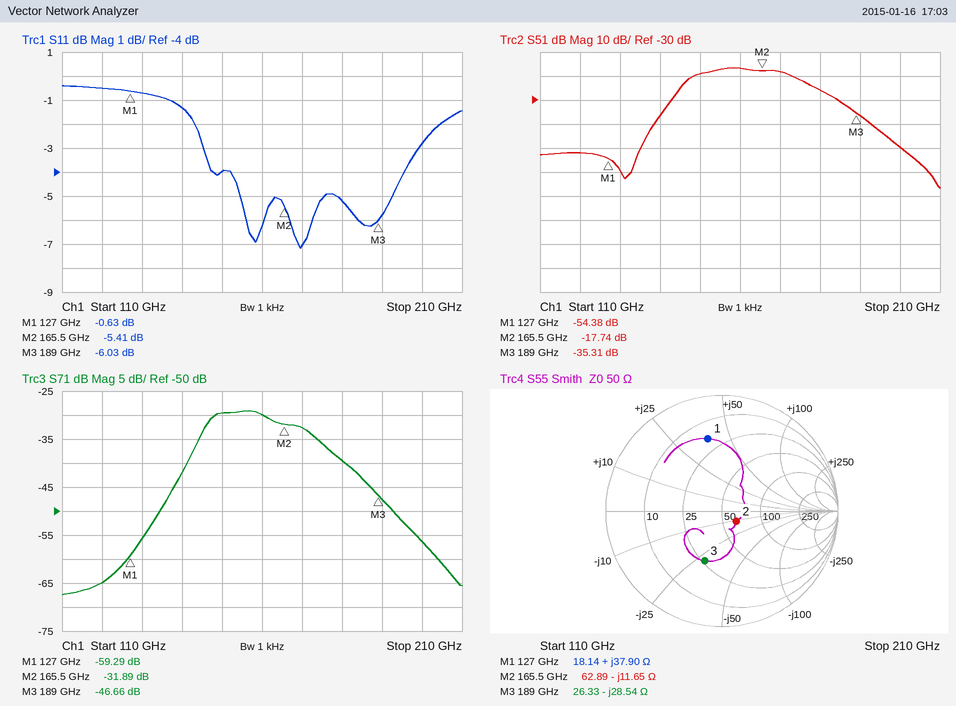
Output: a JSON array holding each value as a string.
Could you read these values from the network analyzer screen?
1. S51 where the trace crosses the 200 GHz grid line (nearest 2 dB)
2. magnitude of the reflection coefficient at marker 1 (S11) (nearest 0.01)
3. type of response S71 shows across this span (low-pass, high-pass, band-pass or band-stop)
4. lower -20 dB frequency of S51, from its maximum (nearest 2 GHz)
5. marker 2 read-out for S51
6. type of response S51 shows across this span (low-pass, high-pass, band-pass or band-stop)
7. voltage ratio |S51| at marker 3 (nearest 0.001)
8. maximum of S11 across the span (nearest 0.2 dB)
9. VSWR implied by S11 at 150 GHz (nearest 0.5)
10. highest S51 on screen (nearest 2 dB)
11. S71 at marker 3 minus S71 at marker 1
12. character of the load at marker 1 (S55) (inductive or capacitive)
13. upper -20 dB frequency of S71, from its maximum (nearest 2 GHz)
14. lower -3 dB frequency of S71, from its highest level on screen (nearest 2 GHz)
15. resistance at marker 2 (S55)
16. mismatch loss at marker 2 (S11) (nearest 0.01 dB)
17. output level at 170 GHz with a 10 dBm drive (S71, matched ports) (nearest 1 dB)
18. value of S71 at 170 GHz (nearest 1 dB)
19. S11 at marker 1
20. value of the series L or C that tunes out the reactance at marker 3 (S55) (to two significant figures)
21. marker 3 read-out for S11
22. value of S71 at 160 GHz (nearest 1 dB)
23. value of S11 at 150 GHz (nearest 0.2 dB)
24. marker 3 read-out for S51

["-50 dB", "0.93", "band-pass", "140 GHz", "-17.74 dB", "band-pass", "0.017", "-0.4 dB", "4.5", "-16 dB", "12.63 dB", "inductive", "192 GHz", "146 GHz", "62.89 Ω", "1.47 dB", "-23 dBm", "-33 dB", "-0.63 dB", "24 pH", "-6.03 dB", "-30 dB", "-4.0 dB", "-35.31 dB"]
